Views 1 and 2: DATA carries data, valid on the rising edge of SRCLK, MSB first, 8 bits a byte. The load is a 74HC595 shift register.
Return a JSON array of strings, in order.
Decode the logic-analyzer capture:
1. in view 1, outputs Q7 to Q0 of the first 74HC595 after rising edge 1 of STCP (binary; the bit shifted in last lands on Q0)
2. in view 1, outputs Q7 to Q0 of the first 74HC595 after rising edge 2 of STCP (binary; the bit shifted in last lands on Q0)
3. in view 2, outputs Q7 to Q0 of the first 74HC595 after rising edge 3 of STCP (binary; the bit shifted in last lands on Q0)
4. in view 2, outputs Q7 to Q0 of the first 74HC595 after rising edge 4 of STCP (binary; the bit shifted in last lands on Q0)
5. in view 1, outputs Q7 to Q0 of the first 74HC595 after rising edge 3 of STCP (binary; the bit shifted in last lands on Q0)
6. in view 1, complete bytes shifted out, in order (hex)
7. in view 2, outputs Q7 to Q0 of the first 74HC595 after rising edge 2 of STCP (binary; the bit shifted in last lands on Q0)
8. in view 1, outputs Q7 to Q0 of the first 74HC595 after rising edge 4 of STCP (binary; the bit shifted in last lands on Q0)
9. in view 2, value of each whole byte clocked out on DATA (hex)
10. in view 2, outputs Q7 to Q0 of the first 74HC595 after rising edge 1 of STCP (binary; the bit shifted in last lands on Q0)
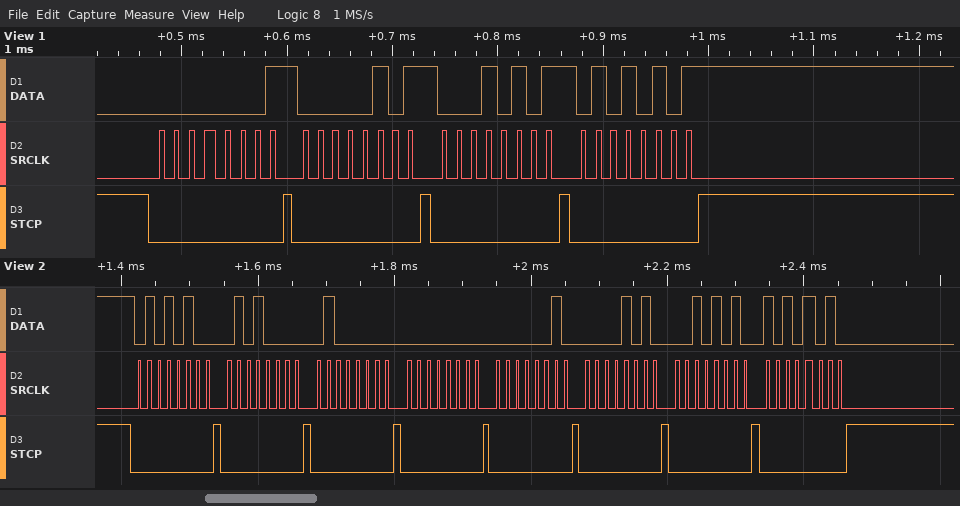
["00000001", "00000101", "01000000", "00000000", "00010101", "01 05 15 55", "01010000", "01010101", "54 50 40 00 02 0A 2A AA", "01010100"]
